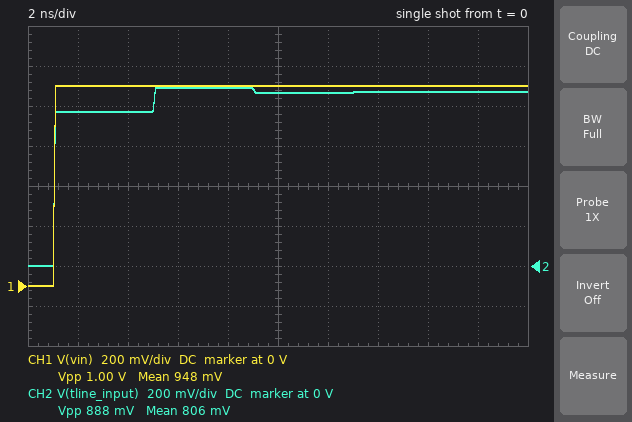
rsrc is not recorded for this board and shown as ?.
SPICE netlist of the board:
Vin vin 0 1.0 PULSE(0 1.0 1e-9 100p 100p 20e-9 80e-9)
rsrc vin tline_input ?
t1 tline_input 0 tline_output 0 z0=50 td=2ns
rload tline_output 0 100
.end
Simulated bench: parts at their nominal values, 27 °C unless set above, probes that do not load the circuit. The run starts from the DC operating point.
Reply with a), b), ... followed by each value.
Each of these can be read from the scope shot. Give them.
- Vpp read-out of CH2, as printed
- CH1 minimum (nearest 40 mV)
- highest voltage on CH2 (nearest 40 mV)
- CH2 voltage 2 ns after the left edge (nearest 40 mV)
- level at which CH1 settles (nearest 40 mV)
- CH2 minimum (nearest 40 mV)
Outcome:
a) 888 mV
b) 0 V
c) 880 mV
d) 760 mV
e) 1.00 V
f) 0 V
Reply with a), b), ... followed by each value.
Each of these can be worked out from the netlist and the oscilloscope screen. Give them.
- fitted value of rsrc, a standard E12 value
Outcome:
a) 15 Ω
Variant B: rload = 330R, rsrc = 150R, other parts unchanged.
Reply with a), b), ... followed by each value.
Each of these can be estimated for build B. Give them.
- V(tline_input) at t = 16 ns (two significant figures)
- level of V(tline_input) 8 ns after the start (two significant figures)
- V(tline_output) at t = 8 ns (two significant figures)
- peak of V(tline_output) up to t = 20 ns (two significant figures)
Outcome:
a) 670 mV
b) 530 mV
c) 590 mV
d) 680 mV
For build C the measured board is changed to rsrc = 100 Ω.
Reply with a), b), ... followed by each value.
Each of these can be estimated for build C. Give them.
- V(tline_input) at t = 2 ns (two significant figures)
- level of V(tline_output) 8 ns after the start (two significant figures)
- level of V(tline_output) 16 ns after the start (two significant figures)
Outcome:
a) 330 mV
b) 490 mV
c) 500 mV
